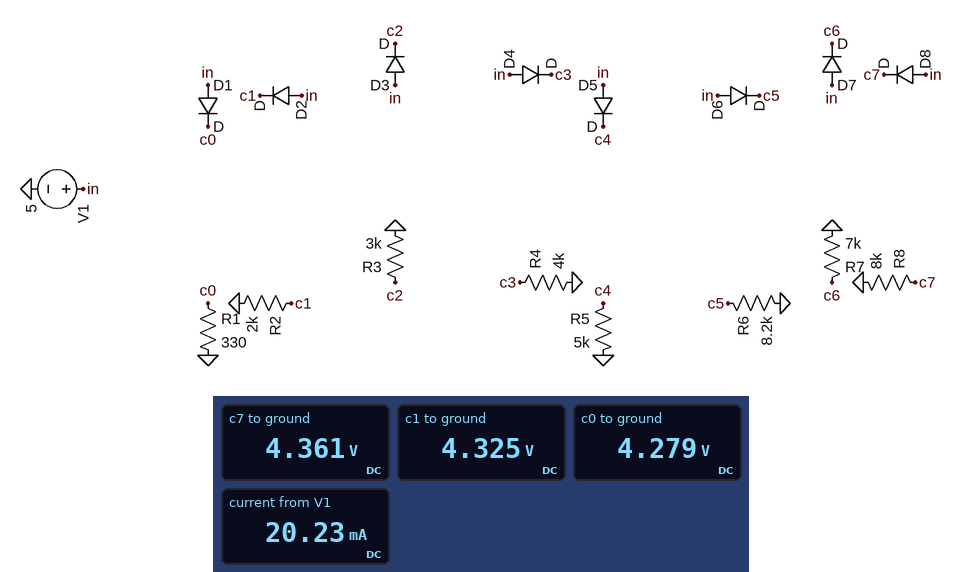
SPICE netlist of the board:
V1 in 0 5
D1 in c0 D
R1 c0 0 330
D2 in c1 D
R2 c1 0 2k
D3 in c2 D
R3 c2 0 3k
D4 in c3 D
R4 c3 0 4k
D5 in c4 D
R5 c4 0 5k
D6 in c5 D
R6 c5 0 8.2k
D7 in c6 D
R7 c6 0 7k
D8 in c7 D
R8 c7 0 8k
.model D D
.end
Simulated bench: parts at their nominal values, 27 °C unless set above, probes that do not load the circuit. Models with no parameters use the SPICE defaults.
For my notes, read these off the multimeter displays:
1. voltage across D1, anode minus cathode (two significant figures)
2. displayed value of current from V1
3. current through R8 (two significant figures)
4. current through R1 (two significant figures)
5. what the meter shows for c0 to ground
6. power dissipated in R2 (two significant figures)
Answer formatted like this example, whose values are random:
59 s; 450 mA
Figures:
720 mV; 20.23 mA; 550 µA; 13 mA; 4.279 V; 9.4 mW
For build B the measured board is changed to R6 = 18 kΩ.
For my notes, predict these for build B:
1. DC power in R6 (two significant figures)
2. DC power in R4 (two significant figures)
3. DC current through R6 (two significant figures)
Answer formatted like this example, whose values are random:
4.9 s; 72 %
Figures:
1.1 mW; 4.7 mW; 240 µA
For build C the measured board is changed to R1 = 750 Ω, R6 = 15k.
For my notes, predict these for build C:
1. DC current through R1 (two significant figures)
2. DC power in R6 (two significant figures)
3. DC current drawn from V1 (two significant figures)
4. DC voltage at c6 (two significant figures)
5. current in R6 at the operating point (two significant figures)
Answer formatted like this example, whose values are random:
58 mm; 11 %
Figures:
5.7 mA; 1.3 mW; 13 mA; 4.4 V; 290 µA
